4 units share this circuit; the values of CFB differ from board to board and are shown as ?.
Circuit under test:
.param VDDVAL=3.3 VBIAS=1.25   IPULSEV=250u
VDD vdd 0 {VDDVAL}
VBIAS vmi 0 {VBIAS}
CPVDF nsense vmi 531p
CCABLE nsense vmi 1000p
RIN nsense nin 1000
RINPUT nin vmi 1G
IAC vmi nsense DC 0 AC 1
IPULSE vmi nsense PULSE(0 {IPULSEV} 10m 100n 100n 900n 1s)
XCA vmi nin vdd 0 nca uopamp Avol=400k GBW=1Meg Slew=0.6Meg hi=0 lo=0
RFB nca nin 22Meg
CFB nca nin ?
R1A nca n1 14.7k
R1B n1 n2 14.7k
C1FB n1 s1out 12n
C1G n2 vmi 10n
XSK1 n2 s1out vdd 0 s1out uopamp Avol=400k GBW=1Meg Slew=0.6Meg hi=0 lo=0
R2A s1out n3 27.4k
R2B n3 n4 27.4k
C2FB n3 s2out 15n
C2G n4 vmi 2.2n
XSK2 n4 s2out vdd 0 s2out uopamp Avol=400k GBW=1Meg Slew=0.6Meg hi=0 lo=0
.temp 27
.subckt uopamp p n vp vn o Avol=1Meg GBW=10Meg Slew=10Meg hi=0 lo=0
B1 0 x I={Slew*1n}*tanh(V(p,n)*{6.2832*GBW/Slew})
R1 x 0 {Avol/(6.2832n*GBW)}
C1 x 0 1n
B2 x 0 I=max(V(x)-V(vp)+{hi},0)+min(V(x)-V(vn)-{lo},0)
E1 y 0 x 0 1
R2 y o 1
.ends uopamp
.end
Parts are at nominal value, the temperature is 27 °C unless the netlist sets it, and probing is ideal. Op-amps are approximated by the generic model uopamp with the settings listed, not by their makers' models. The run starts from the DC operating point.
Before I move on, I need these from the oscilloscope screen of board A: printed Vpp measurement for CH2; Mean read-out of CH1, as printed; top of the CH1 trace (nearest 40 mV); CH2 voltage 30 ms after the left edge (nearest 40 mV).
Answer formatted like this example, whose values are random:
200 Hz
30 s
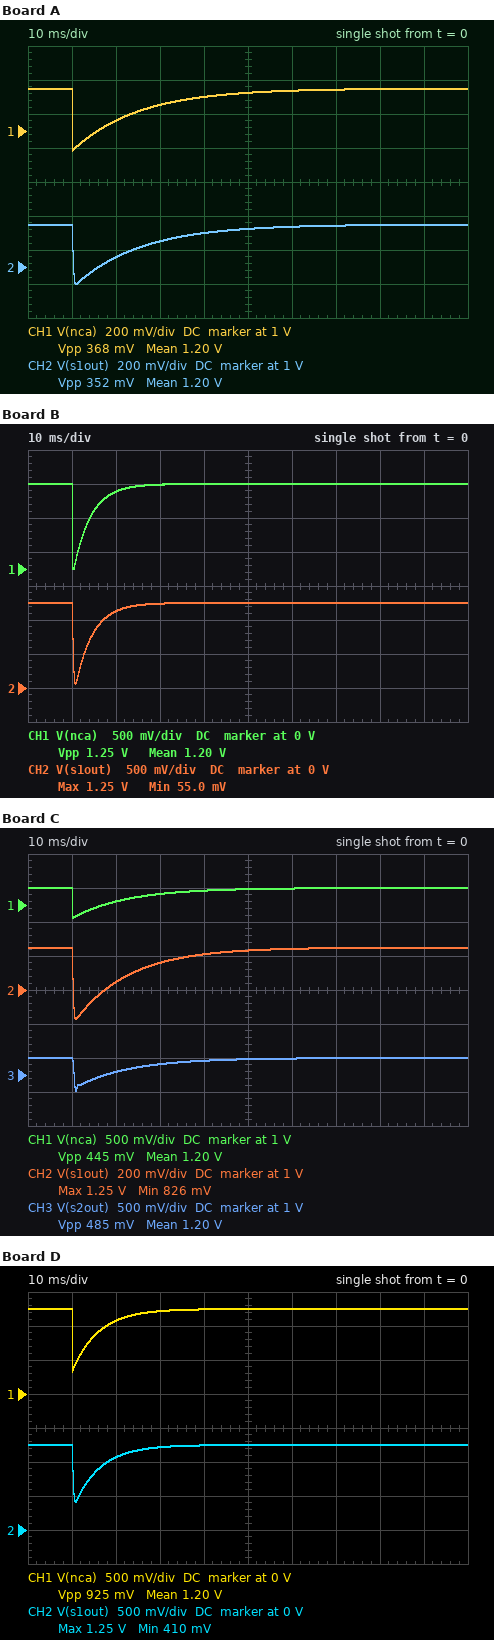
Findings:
352 mV
1.20 V
1.24 V
1.16 V
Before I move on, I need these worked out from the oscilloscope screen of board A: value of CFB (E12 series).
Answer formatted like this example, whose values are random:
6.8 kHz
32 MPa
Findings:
680 pF
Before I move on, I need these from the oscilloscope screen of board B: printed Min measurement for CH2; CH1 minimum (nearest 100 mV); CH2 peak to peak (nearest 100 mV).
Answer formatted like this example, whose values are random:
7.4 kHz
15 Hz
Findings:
55.0 mV
0 V
1.2 V
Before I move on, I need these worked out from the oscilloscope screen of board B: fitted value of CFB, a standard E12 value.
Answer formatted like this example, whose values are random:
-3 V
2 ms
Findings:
180 pF
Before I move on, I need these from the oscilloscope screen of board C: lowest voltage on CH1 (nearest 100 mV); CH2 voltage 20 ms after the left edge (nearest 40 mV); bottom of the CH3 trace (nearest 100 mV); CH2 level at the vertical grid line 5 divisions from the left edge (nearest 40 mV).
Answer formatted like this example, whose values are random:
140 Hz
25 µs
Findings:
800 mV
1.04 V
800 mV
1.24 V
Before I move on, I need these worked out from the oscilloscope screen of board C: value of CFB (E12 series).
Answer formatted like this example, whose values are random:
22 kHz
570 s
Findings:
560 pF
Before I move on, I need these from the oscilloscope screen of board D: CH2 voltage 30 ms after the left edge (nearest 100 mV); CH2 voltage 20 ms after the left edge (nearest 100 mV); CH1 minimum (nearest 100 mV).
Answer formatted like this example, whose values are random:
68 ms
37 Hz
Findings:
1.2 V
1.1 V
300 mV
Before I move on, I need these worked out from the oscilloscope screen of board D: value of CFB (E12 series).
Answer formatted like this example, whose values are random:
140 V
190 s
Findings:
270 pF
